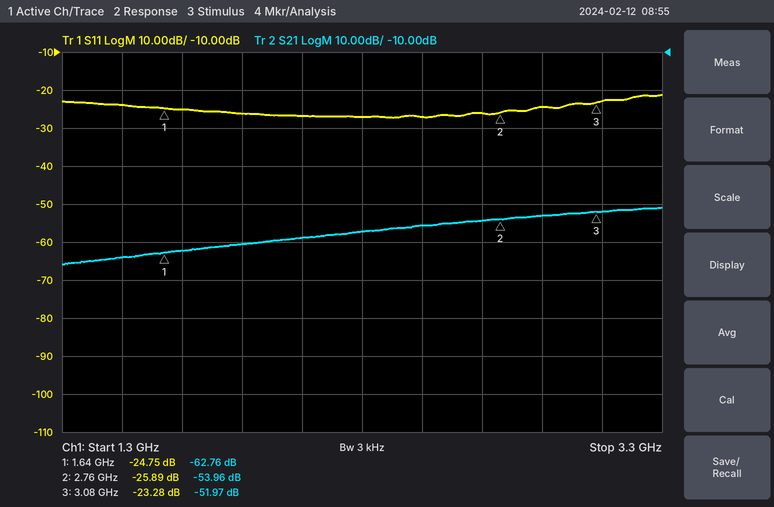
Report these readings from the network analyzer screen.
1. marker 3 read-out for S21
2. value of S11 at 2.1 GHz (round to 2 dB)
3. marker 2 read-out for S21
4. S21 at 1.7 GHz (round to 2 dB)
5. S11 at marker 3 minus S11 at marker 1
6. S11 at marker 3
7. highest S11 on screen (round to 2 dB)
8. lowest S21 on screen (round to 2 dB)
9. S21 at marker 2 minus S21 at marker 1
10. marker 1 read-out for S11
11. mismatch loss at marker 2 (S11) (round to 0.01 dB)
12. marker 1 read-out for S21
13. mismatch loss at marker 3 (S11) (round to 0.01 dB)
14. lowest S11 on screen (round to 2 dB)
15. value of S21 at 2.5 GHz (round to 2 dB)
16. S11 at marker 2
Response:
-51.97 dB
-26 dB
-53.96 dB
-62 dB
1.47 dB
-23.28 dB
-22 dB
-66 dB
8.80 dB
-24.75 dB
0.01 dB
-62.76 dB
0.02 dB
-28 dB
-56 dB
-25.89 dB
